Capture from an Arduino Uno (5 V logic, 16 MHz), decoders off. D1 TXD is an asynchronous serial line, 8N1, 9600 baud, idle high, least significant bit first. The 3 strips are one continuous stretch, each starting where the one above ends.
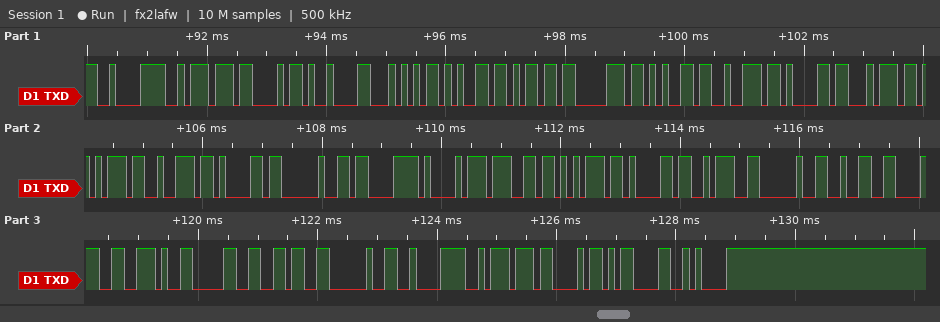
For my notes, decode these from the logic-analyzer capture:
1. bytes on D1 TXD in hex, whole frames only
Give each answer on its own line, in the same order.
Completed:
C2 BA 43 09 54 65 6D 70 65 72 61 74 75 72 61 20 C3 A1 67 75 61 3A 20 32 38 2E 30 36 20 C2 BA 43 0D 0A
